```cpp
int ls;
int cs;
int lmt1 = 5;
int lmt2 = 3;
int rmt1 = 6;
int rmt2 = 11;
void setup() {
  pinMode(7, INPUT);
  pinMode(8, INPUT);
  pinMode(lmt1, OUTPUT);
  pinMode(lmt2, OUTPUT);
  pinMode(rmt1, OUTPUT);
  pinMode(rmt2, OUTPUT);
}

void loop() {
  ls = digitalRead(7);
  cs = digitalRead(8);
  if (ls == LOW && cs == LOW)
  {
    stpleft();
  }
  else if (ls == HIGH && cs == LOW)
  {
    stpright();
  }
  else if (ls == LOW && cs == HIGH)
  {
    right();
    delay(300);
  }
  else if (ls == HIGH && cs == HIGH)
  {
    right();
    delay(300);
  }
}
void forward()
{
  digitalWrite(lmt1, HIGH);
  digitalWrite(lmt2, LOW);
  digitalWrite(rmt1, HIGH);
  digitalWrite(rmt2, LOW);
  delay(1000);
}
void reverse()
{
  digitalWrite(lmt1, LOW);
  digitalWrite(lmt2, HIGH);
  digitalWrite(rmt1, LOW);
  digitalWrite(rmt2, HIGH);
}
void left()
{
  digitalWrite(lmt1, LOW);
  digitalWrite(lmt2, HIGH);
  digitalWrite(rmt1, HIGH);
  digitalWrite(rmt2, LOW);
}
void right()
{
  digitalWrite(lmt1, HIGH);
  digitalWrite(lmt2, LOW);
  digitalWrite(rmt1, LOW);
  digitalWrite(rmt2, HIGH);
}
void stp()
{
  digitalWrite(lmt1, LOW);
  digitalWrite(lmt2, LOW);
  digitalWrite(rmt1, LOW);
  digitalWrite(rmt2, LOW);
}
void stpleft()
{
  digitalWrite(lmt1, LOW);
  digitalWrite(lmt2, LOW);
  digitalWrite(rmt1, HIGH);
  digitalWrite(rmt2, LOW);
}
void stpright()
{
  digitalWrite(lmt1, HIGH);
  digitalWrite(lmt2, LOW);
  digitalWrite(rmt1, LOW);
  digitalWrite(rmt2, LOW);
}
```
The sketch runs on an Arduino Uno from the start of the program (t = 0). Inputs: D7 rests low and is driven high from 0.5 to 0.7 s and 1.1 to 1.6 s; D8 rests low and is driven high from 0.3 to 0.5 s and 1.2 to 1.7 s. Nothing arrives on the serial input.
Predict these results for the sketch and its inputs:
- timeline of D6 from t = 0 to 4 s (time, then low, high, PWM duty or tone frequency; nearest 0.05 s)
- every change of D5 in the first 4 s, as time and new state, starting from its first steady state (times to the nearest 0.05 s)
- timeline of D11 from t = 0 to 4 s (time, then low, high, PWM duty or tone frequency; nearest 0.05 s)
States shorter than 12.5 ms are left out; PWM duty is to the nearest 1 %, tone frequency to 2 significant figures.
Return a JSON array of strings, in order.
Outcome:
["0 s high; 0.3 s low; 0.7 s high; 1.1 s low; 1.8 s high", "0 s low; 0.3 s high; 0.7 s low; 1.1 s high; 1.8 s low", "0 s low; 0.3 s high; 0.6 s low; 1.2 s high; 1.8 s low"]
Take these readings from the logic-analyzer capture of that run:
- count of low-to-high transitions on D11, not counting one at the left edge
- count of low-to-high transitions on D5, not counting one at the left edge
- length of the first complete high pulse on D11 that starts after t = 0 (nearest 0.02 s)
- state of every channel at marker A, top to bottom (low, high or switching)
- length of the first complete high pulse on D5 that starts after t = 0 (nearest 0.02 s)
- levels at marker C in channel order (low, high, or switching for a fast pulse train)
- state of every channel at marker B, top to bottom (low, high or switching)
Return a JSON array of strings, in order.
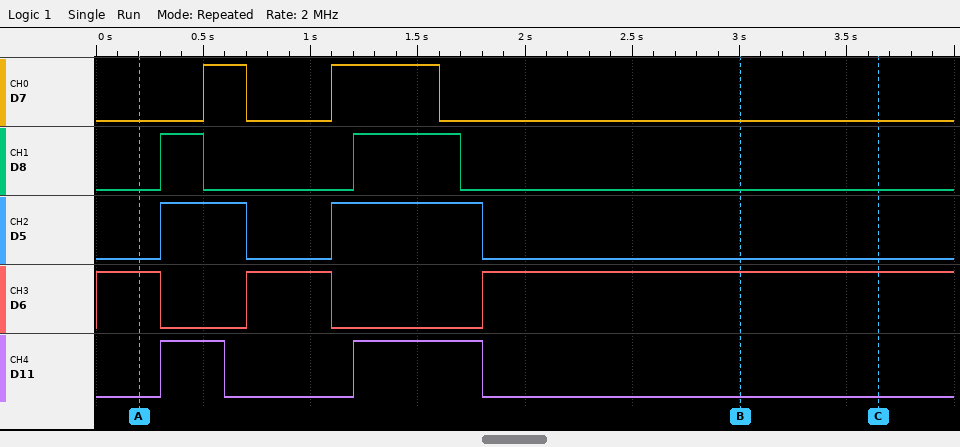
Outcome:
["2", "2", "0.30 s", "D7 low, D8 low, D5 low, D6 high, D11 low", "0.40 s", "D7 low, D8 low, D5 low, D6 high, D11 low", "D7 low, D8 low, D5 low, D6 high, D11 low"]
